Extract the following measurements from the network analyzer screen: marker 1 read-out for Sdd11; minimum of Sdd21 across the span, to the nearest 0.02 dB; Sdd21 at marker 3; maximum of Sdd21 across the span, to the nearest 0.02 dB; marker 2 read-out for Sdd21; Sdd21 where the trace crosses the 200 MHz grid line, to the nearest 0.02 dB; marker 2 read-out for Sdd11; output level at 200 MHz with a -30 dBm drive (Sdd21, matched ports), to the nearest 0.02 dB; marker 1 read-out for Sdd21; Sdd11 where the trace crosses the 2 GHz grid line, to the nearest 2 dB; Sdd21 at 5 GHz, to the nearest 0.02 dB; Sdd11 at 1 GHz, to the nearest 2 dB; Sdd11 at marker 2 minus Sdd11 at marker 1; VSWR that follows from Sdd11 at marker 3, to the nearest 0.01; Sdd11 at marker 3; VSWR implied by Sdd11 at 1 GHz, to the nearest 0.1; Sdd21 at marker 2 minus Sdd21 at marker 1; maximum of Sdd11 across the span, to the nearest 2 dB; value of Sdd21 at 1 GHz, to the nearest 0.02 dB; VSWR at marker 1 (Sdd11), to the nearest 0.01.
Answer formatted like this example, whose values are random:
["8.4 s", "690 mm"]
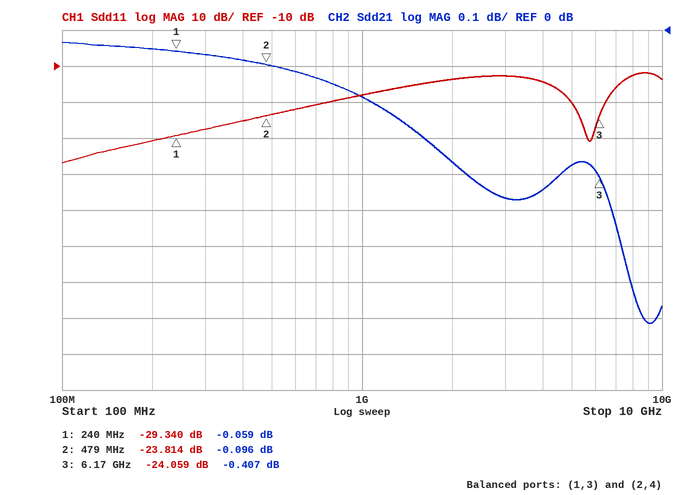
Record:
["-29.340 dB", "-0.82 dB", "-0.407 dB", "-0.04 dB", "-0.096 dB", "-0.06 dB", "-23.814 dB", "-30.06 dBm", "-0.059 dB", "-14 dB", "-0.38 dB", "-18 dB", "5.526 dB", "1.13", "-24.059 dB", "1.3", "-0.037 dB", "-12 dB", "-0.18 dB", "1.07"]
